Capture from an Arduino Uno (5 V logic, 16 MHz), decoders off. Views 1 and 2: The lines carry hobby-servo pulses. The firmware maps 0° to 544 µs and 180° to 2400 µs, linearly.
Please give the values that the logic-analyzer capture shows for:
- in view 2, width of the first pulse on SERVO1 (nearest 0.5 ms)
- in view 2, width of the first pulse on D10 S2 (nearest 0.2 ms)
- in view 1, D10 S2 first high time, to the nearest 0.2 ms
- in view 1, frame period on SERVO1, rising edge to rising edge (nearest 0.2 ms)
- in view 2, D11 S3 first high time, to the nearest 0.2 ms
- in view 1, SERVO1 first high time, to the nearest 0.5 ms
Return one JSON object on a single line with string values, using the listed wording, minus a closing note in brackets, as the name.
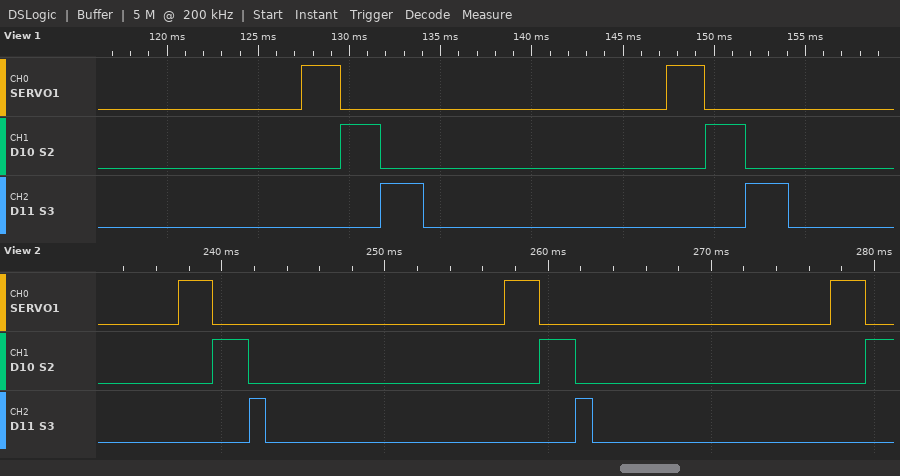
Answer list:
{"in view 2, width of the first pulse on SERVO1": "2.0 ms", "in view 2, width of the first pulse on D10 S2": "2.2 ms", "in view 1, D10 S2 first high time, to the nearest 0.2 ms": "2.2 ms", "in view 1, frame period on SERVO1, rising edge to rising edge": "20.0 ms", "in view 2, D11 S3 first high time, to the nearest 0.2 ms": "1.0 ms", "in view 1, SERVO1 first high time, to the nearest 0.5 ms": "2.0 ms"}
